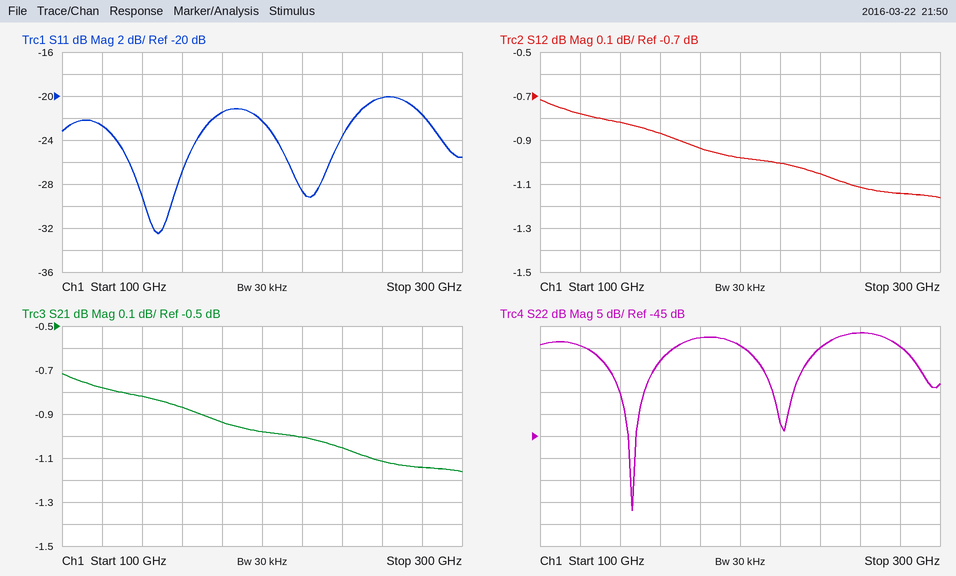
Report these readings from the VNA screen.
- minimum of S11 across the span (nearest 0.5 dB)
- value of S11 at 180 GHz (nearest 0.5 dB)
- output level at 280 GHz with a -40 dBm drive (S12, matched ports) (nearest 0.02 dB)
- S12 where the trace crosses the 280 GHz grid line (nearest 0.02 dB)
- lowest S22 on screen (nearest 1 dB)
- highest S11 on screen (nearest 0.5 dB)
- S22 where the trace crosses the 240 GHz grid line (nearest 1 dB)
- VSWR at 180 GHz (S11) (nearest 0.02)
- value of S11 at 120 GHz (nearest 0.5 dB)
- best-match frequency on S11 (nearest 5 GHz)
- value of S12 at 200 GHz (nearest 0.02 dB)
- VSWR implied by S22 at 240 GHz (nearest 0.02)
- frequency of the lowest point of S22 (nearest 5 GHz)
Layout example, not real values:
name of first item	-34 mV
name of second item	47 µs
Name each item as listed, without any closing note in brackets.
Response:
minimum of S11 across the span	-32.5 dB
value of S11 at 180 GHz	-21.5 dB
output level at 280 GHz with a -40 dBm drive (S12, matched ports)	-41.14 dBm
S12 where the trace crosses the 280 GHz grid line	-1.14 dB
lowest S22 on screen	-62 dB
highest S11 on screen	-20.0 dB
S22 where the trace crosses the 240 GHz grid line	-25 dB
VSWR at 180 GHz (S11)	1.18
value of S11 at 120 GHz	-22.5 dB
best-match frequency on S11	150 GHz
value of S12 at 200 GHz	-0.98 dB
VSWR implied by S22 at 240 GHz	1.12
frequency of the lowest point of S22	145 GHz
